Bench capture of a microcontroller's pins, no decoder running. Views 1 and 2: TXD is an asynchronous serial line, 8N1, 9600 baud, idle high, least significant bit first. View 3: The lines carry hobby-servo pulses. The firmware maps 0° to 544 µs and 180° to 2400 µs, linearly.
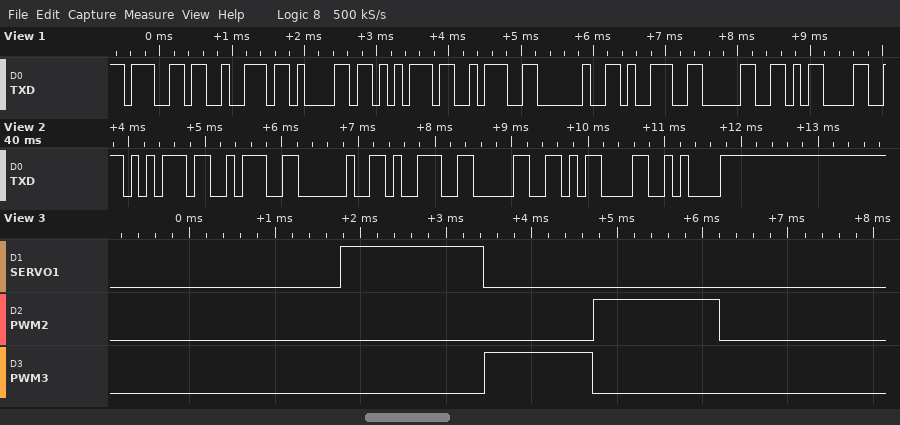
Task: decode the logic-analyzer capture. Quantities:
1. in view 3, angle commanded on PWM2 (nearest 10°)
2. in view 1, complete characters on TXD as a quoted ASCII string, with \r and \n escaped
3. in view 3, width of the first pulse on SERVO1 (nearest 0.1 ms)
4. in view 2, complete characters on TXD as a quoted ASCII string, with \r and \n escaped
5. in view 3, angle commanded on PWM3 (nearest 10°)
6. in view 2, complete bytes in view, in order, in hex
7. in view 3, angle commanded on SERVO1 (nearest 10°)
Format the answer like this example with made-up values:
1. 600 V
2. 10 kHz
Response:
1. 90°
2. "grau: 90\r"
3. 1.7 ms
4. "u: 90\r\n"
5. 70°
6. 75 3A 20 39 30 0D 0A
7. 110°
